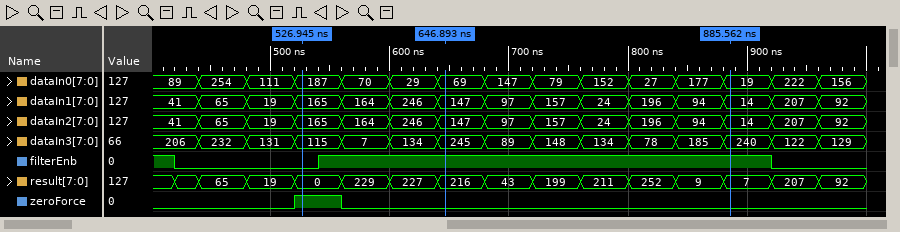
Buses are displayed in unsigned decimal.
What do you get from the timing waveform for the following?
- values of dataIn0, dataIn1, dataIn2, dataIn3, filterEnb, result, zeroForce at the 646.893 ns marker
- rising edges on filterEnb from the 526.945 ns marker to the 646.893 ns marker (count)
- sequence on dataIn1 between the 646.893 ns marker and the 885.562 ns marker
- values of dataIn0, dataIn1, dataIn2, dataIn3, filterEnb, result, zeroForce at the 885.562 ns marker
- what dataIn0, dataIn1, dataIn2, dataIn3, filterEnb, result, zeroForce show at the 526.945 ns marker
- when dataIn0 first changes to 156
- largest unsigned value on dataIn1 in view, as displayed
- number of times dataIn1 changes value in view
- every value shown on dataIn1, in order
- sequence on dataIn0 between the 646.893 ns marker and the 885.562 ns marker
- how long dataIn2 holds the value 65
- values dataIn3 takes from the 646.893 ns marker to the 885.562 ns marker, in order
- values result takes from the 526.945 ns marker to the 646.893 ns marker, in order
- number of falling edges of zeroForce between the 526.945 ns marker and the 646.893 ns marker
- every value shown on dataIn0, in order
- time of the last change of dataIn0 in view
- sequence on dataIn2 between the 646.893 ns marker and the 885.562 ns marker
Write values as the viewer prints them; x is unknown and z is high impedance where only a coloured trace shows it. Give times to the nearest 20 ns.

dataIn0=69, dataIn1=147, dataIn2=147, dataIn3=245, filterEnb=1, result=216, zeroForce=0
1
147, 97, 157, 24, 196, 94, 14
dataIn0=19, dataIn1=14, dataIn2=14, dataIn3=240, filterEnb=1, result=7, zeroForce=0
dataIn0=187, dataIn1=165, dataIn2=165, dataIn3=115, filterEnb=0, result=0, zeroForce=1
960 ns
246
14
41, 65, 19, 165, 164, 246, 147, 97, 157, 24, 196, 94, 14, 207, 92
69, 147, 79, 152, 27, 177, 19
40 ns
245, 89, 148, 134, 78, 185, 240
0, 229, 227, 216
1
89, 254, 111, 187, 70, 29, 69, 147, 79, 152, 27, 177, 19, 222, 156
960 ns
147, 97, 157, 24, 196, 94, 14
